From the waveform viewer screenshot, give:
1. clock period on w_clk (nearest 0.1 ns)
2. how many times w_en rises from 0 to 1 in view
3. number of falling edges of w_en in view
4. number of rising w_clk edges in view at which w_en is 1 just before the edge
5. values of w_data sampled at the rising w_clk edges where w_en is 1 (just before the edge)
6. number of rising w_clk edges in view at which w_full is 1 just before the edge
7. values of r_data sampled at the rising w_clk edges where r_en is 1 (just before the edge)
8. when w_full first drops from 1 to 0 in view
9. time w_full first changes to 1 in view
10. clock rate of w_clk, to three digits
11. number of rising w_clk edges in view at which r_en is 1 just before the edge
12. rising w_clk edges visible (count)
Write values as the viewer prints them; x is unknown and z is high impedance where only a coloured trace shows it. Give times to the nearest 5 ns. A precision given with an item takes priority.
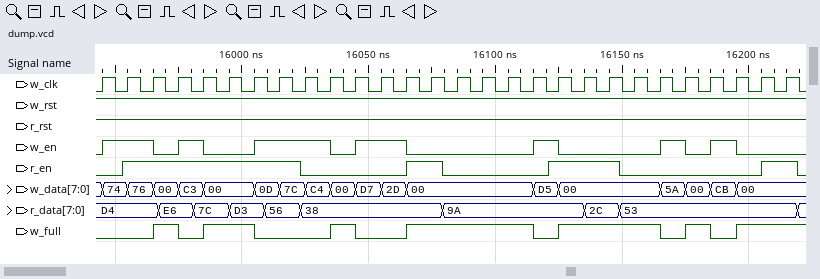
10 ns
7
7
11
74, 76, C3, 0D, 7C, C4, D7, 2D, D5, 5A, CB
16
D4, D4, E6, 7C, 7C, D3, 56, 38, 9A, 9A, 2C, 53
15975 ns
15965 ns
100 MHz
12
28
